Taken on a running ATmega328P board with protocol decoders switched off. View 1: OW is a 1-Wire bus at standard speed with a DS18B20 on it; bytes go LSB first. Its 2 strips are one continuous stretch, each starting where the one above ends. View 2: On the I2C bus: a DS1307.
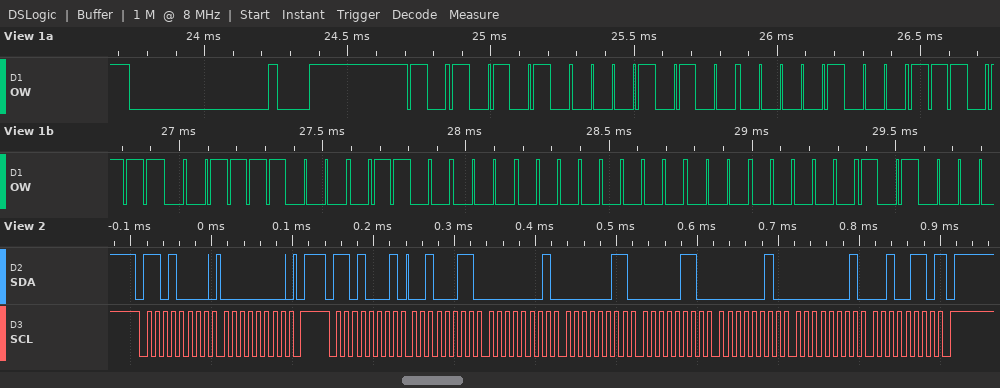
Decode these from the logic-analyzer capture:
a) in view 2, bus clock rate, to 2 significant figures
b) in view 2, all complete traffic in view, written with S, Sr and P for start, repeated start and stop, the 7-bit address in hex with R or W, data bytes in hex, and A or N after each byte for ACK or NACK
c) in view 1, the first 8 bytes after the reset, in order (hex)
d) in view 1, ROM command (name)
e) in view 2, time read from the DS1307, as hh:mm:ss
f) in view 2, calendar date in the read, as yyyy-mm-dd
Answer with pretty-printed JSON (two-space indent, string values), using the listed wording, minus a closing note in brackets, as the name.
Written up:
{
  "in view 2, bus clock rate, to 2 significant figures": "100 kHz",
  "in view 2, all complete traffic in view, written with S, Sr and P for start, repeated start and stop, the 7-bit address in hex with R or W, data bytes in hex, and A or N after each byte for ACK or NACK": "S 68W A 00 A P S 68R A 23 A 01 A 03 A 06 A 02 A 01 A 26 N P",
  "in view 1, the first 8 bytes after the reset, in order": "55 28 10 77 1E 06 00 00",
  "in view 1, ROM command": "Match ROM",
  "in view 2, time read from the DS1307, as hh:mm:ss": "03:01:23",
  "in view 2, calendar date in the read, as yyyy-mm-dd": "2026-01-02"
}
